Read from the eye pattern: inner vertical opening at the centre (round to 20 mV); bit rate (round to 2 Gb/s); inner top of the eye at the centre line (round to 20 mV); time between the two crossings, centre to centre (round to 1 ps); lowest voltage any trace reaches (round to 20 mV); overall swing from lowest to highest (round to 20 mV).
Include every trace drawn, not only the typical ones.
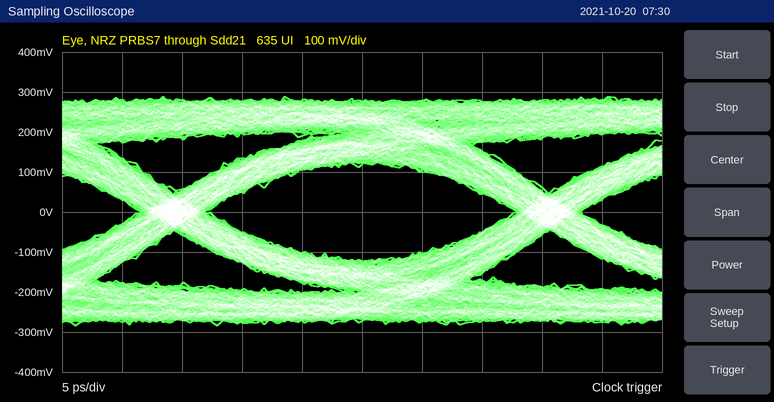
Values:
240 mV
32 Gb/s
120 mV
31 ps
-280 mV
580 mV
